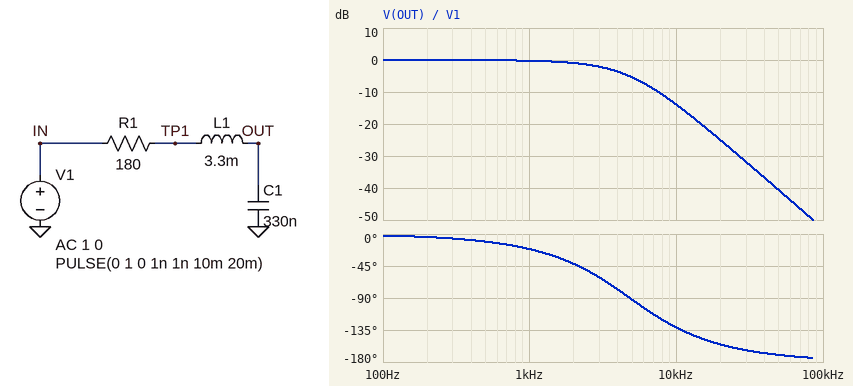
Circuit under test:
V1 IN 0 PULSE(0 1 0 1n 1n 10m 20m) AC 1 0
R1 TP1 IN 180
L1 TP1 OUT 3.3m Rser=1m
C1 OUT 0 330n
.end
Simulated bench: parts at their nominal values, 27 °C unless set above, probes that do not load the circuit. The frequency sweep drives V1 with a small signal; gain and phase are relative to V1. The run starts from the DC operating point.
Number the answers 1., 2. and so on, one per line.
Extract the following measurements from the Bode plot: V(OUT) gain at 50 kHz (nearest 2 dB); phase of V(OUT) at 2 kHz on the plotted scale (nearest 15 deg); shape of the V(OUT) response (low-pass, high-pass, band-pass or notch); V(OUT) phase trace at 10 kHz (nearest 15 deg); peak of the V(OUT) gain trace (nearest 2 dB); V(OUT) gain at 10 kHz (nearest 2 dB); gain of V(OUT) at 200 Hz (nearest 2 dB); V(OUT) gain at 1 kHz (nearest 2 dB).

1. -40 dB
2. -45 deg
3. low-pass
4. -135 deg
5. 0 dB
6. -14 dB
7. 0 dB
8. 0 dB
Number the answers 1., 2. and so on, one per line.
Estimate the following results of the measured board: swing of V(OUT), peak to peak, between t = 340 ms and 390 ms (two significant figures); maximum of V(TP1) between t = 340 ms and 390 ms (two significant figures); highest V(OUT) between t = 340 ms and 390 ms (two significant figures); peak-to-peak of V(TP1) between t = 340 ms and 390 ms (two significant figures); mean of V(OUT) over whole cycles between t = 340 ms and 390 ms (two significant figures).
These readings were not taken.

1. 1.0 V
2. 1.0 V
3. 1.0 V
4. 1.0 V
5. 500 mV
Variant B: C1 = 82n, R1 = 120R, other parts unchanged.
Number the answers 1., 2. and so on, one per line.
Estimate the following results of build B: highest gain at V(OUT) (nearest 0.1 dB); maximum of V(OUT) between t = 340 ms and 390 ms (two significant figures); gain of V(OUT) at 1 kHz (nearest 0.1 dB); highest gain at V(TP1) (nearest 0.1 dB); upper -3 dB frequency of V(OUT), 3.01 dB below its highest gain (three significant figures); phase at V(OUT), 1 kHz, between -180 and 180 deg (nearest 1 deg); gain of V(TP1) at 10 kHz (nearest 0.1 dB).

1. 4.9 dB
2. 1.4 V
3. 0.1 dB
4. 0 dB
5. 11.4 kHz
6. -4 deg
7. -19.2 dB
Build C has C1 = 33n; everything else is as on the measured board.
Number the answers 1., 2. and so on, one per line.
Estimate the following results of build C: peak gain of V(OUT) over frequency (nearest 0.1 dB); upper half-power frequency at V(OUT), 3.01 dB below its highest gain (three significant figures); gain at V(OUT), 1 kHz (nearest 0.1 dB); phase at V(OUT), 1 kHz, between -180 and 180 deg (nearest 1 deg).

1. 5.3 dB
2. 17.9 kHz
3. 0 dB
4. -2 deg
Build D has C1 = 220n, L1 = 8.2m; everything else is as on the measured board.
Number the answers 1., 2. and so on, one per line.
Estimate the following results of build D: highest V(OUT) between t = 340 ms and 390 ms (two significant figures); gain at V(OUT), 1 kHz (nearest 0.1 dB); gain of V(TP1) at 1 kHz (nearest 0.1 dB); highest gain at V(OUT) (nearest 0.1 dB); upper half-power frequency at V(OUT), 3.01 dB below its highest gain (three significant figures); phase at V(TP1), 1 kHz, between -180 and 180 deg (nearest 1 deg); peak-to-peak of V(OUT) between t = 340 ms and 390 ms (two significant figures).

1. 1.2 V
2. 0.3 dB
3. -0.3 dB
4. 1.7 dB
5. 4.42 kHz
6. -15 deg
7. 1.4 V
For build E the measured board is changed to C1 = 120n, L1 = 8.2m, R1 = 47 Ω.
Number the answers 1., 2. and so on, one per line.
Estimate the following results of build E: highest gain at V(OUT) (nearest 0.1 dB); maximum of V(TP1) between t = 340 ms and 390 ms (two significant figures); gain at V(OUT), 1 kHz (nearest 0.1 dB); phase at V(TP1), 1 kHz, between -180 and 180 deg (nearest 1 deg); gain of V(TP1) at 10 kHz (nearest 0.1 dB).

1. 14.9 dB
2. 1.1 V
3. 0.3 dB
4. -2 deg
5. -0.1 dB
